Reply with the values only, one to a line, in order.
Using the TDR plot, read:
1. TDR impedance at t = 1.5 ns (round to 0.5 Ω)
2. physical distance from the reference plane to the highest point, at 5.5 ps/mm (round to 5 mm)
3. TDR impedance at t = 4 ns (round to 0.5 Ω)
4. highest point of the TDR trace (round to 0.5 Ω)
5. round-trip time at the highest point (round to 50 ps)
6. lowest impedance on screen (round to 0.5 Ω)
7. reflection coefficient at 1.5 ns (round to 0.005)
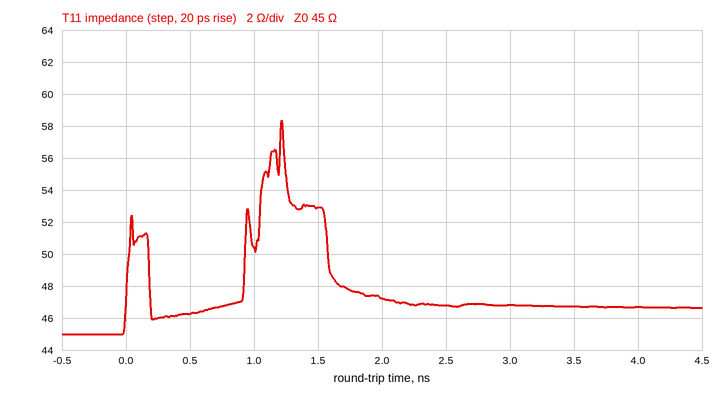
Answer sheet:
53.0 Ω
110 mm
46.5 Ω
58.5 Ω
1.20 ns
45.0 Ω
+0.080
